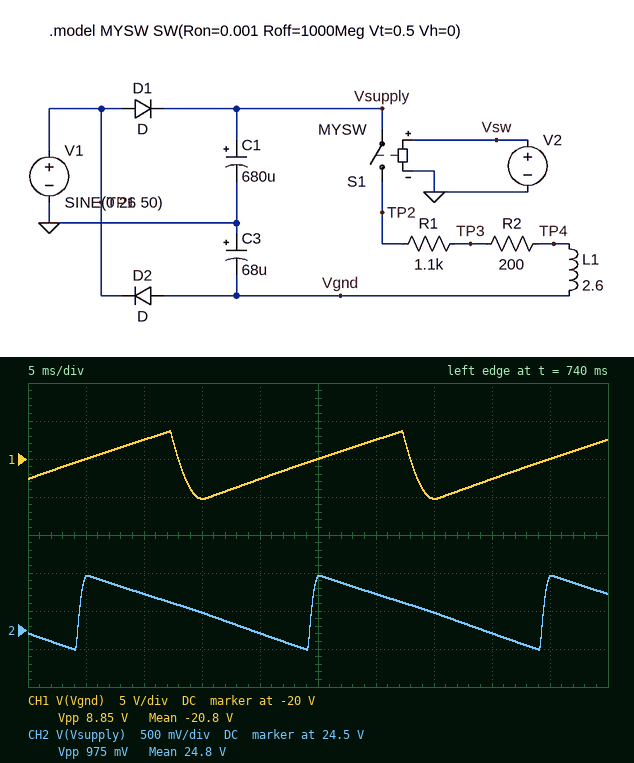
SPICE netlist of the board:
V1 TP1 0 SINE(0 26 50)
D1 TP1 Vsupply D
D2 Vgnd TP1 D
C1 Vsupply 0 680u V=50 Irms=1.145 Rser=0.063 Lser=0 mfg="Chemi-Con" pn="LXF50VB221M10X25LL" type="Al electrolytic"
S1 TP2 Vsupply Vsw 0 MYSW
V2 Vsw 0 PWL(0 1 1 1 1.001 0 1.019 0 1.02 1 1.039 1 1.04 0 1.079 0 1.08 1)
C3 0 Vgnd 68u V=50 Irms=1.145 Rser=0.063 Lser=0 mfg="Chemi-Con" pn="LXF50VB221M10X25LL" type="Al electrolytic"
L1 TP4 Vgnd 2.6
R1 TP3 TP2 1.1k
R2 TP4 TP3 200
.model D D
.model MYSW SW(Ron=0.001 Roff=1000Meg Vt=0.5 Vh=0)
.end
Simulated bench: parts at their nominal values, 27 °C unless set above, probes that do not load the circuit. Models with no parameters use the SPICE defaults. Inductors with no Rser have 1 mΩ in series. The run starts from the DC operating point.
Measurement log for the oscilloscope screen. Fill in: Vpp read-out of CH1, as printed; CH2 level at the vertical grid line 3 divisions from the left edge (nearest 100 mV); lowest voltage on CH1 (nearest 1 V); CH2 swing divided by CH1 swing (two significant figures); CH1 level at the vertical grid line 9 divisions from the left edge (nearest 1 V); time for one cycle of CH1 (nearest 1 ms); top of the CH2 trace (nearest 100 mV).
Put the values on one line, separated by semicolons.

8.85 V; 24.7 V; -25 V; 0.11; -20 V; 20 ms; 25.2 V
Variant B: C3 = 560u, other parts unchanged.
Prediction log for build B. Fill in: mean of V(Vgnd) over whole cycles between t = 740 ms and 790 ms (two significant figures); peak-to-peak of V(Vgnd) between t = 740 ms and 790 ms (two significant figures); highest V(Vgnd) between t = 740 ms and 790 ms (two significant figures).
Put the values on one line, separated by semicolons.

-25 V; 1.3 V; -24 V
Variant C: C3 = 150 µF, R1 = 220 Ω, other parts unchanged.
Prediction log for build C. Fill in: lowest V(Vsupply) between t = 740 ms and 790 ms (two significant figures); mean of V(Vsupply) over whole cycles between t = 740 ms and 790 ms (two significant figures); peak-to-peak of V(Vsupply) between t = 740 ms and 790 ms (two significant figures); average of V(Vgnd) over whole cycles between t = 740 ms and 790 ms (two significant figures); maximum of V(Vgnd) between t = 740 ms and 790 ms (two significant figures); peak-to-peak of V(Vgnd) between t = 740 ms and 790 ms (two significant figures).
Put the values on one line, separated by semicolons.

22 V; 24 V; 2.8 V; -20 V; -14 V; 12 V
